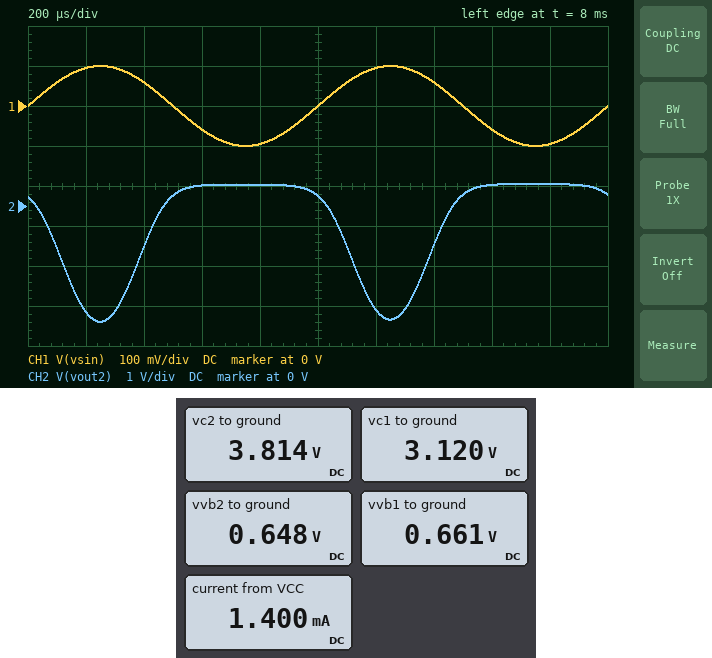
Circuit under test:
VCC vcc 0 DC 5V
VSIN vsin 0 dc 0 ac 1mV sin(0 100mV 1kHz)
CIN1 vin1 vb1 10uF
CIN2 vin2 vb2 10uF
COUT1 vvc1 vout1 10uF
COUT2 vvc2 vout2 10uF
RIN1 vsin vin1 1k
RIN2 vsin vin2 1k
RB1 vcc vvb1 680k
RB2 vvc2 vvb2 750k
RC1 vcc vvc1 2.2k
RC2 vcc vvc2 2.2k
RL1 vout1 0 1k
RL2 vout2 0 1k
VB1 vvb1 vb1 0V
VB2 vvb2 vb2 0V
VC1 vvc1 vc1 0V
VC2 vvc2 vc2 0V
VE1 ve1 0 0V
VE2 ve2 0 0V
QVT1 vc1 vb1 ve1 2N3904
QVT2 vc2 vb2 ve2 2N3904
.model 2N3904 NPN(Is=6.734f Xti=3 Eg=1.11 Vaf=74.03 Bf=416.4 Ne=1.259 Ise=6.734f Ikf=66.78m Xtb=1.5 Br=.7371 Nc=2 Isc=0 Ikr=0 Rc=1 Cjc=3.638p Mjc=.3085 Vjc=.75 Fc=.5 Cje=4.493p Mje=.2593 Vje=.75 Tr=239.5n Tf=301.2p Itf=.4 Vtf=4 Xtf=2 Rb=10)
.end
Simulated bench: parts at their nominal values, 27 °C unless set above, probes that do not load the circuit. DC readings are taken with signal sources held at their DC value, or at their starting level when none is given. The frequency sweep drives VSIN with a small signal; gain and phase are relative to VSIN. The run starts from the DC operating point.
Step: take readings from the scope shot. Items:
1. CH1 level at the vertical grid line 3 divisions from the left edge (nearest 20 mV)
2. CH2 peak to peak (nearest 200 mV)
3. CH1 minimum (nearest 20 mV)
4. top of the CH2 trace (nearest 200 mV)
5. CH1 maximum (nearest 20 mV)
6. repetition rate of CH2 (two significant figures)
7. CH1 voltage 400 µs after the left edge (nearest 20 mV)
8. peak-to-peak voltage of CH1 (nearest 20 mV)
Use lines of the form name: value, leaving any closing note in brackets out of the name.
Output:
CH1 level at the vertical grid line 3 divisions from the left edge: -60 mV
CH2 peak to peak: 3.4 V
CH1 minimum: -100 mV
top of the CH2 trace: 600 mV
CH1 maximum: 100 mV
repetition rate of CH2: 1.0 kHz
CH1 voltage 400 µs after the left edge: 60 mV
peak-to-peak voltage of CH1: 200 mV
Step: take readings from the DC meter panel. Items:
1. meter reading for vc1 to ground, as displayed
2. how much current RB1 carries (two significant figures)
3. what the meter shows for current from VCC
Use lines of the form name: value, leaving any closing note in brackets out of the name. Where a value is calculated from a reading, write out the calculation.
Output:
meter reading for vc1 to ground, as displayed: 3.120 V
how much current RB1 carries: (5 V - 661 mV) / 680 kΩ = 6.4 µA
what the meter shows for current from VCC: 1.400 mA
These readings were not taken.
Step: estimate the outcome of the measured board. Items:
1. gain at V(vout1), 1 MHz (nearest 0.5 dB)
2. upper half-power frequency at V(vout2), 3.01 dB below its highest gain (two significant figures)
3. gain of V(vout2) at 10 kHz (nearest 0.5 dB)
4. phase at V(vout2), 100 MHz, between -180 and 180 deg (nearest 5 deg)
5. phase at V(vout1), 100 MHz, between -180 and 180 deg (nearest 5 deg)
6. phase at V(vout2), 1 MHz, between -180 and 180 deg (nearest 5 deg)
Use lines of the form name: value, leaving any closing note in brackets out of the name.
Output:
gain at V(vout1), 1 MHz: 24.5 dB
upper half-power frequency at V(vout2), 3.01 dB below its highest gain: 3.9 MHz
gain of V(vout2) at 10 kHz: 21.5 dB
phase at V(vout2), 100 MHz, between -180 and 180 deg: 75 deg
phase at V(vout1), 100 MHz, between -180 and 180 deg: 75 deg
phase at V(vout2), 1 MHz, between -180 and 180 deg: 165 deg
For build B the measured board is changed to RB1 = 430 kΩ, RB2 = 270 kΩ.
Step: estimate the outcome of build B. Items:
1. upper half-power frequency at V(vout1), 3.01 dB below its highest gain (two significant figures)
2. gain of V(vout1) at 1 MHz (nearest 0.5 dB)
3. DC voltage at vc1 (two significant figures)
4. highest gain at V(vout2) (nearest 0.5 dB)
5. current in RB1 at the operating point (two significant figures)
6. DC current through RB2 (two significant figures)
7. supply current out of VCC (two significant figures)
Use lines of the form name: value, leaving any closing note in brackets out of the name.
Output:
upper half-power frequency at V(vout1), 3.01 dB below its highest gain: 1.7 MHz
gain of V(vout1) at 1 MHz: 27.5 dB
DC voltage at vc1: 1.9 V
highest gain at V(vout2): 26.0 dB
current in RB1 at the operating point: 10 µA
DC current through RB2: 7.6 µA
supply current out of VCC: 2.5 mA
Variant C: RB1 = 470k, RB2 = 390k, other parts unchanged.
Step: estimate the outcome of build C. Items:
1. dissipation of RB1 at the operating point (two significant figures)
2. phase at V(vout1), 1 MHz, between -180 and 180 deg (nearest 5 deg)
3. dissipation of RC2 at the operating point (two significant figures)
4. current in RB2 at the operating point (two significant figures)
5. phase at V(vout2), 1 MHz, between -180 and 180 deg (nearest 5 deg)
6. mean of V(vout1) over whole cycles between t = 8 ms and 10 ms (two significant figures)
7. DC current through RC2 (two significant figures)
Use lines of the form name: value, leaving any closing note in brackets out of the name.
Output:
dissipation of RB1 at the operating point: 40 µW
phase at V(vout1), 1 MHz, between -180 and 180 deg: 150 deg
dissipation of RC2 at the operating point: 1.6 mW
current in RB2 at the operating point: 6.3 µA
phase at V(vout2), 1 MHz, between -180 and 180 deg: 160 deg
mean of V(vout1) over whole cycles between t = 8 ms and 10 ms: -200 mV
DC current through RC2: 850 µA
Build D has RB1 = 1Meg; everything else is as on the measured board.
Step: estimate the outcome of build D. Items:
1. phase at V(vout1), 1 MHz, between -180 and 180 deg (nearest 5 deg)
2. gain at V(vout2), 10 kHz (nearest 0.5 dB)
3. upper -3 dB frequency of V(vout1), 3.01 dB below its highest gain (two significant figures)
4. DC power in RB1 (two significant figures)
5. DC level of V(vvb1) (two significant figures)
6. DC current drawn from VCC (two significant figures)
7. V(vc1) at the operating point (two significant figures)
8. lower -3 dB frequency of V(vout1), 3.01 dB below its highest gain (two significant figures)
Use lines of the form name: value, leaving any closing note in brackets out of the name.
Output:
phase at V(vout1), 1 MHz, between -180 and 180 deg: 165 deg
gain at V(vout2), 10 kHz: 21.5 dB
upper -3 dB frequency of V(vout1), 3.01 dB below its highest gain: 3.8 MHz
DC power in RB1: 19 µW
DC level of V(vvb1): 650 mV
DC current drawn from VCC: 1.1 mA
V(vc1) at the operating point: 3.8 V
lower -3 dB frequency of V(vout1), 3.01 dB below its highest gain: 5.7 Hz
